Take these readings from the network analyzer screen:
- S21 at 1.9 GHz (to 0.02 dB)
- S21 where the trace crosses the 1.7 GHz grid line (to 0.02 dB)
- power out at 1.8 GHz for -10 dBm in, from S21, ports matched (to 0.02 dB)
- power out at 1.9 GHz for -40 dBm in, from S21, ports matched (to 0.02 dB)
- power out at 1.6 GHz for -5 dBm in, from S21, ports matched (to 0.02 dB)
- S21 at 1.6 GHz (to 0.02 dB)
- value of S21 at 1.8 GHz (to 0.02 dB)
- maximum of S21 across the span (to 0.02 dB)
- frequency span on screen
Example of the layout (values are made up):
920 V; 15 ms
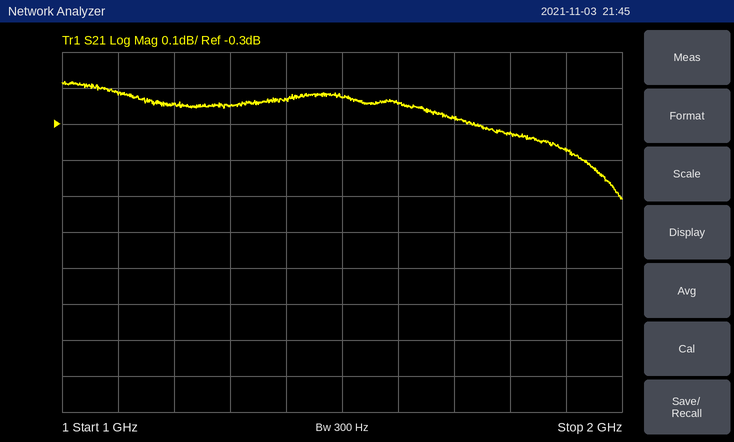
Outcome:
-0.38 dB; -0.28 dB; -10.32 dBm; -40.38 dBm; -5.24 dBm; -0.24 dB; -0.32 dB; -0.18 dB; 1 GHz
